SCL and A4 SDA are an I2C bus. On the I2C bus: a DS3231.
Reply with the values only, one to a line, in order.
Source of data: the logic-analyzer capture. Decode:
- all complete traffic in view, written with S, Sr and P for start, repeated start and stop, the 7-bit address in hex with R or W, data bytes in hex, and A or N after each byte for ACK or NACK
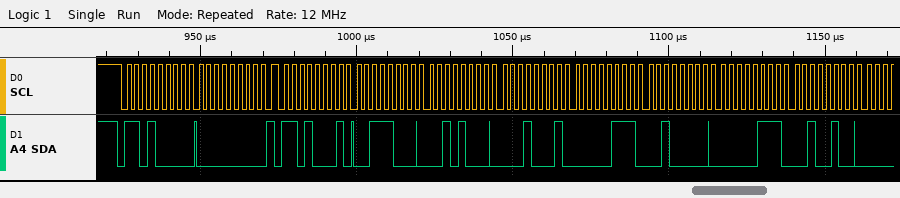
S 68W A 00 A Sr 68R A 38 A 28 A 11 A 07 A 20 A 07 A 24 A
